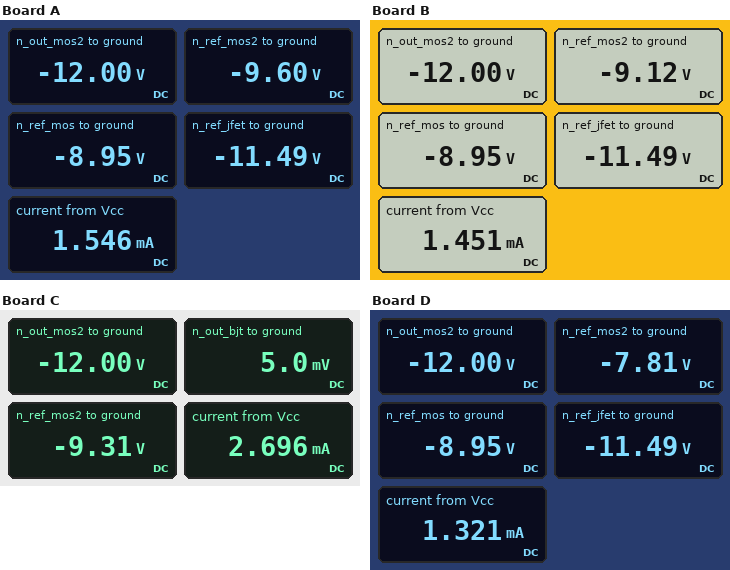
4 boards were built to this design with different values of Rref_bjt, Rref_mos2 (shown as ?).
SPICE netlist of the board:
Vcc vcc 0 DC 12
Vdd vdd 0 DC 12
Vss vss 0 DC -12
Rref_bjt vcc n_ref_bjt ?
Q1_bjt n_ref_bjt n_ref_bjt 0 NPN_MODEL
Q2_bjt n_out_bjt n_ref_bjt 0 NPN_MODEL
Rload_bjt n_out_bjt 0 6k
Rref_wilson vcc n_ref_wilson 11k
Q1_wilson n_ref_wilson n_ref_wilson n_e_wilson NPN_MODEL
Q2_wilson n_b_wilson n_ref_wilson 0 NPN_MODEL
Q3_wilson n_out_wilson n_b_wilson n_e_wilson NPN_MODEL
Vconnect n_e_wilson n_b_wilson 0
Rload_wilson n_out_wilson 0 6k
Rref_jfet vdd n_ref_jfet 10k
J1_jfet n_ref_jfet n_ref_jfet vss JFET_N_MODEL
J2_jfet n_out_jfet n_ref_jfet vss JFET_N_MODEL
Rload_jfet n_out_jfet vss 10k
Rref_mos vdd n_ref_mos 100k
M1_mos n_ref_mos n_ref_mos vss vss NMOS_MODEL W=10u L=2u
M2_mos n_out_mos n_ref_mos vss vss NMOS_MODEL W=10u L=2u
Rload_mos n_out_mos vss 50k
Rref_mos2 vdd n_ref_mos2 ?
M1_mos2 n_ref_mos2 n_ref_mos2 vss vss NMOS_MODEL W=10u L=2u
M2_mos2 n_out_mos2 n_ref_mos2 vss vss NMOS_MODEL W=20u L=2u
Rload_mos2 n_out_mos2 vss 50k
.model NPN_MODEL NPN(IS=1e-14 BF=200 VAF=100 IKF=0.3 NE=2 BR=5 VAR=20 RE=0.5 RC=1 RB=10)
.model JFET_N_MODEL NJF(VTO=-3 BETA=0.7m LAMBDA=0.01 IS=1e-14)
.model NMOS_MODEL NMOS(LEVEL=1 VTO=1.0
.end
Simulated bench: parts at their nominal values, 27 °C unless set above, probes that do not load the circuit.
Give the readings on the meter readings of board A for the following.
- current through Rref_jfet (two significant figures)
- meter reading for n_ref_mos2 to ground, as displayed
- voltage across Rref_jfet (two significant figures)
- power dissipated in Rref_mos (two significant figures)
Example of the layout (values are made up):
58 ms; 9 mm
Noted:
2.3 mA; -9.60 V; 23 V; 4.4 mW
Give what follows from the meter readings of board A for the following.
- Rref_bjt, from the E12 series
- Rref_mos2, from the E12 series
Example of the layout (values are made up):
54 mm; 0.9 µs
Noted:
22 kΩ; 220 kΩ
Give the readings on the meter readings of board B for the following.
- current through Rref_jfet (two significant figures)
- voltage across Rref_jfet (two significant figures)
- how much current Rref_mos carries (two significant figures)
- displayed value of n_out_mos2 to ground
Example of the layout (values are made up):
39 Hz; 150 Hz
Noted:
2.3 mA; 23 V; 210 µA; -12.00 V
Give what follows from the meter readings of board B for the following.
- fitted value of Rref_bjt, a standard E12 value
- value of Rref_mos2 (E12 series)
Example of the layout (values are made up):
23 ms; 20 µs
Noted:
27 kΩ; 120 kΩ
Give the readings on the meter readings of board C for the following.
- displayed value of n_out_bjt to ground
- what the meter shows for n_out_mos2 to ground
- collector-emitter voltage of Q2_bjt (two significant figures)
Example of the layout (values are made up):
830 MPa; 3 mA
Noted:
5.0 mV; -12.00 V; 5.0 mV
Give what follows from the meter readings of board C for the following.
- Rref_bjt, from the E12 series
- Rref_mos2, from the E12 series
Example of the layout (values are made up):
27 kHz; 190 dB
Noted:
6.8 kΩ; 150 kΩ
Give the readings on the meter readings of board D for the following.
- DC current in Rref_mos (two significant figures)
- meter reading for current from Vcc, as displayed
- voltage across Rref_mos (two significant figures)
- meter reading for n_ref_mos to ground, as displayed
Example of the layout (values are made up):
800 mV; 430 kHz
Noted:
210 µA; 1.321 mA; 21 V; -8.95 V
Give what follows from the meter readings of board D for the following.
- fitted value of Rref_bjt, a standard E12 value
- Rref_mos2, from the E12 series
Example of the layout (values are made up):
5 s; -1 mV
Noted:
39 kΩ; 39 kΩ
